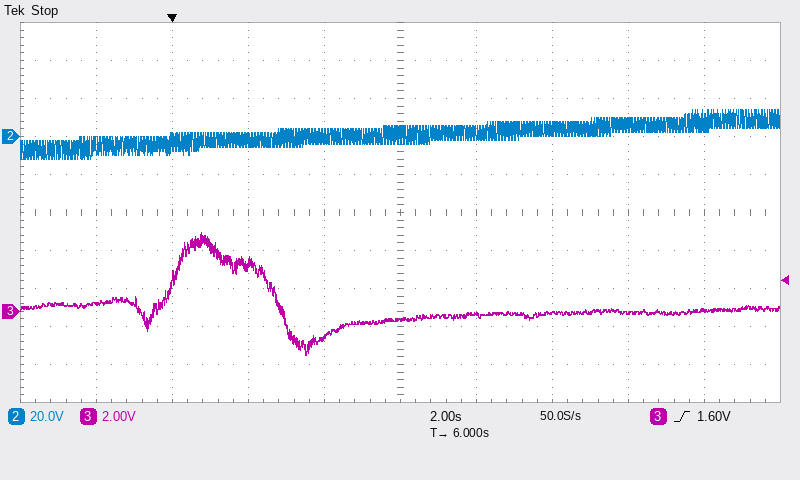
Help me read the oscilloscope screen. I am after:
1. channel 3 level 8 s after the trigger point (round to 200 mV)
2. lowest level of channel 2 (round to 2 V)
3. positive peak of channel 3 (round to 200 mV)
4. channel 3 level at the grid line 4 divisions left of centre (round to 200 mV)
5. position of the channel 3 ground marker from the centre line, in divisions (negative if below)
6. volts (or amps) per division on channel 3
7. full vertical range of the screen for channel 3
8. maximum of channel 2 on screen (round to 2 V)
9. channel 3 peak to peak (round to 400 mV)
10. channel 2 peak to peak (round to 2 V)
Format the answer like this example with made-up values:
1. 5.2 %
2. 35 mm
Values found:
1. -200 mV
2. -12 V
3. 4.2 V
4. 400 mV
5. -2.6 div
6. 2 V
7. 20 V
8. 14 V
9. 6.4 V
10. 26 V
